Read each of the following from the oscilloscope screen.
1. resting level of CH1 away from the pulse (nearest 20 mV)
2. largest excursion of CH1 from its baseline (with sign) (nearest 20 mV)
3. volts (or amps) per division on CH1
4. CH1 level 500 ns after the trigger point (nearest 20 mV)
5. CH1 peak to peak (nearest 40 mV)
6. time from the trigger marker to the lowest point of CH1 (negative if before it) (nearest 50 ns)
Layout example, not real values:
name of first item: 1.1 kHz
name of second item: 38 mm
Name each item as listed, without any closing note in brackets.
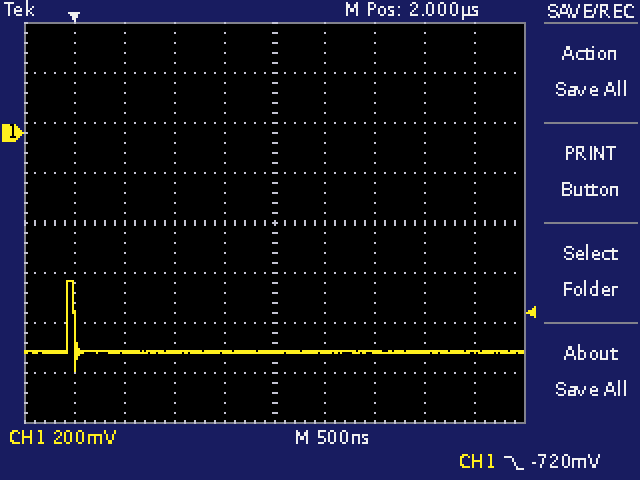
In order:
resting level of CH1 away from the pulse: -880 mV
largest excursion of CH1 from its baseline (with sign): +280 mV
volts (or amps) per division on CH1: 200 mV
CH1 level 500 ns after the trigger point: -880 mV
CH1 peak to peak: 360 mV
time from the trigger marker to the lowest point of CH1 (negative if before it): 0 ns
